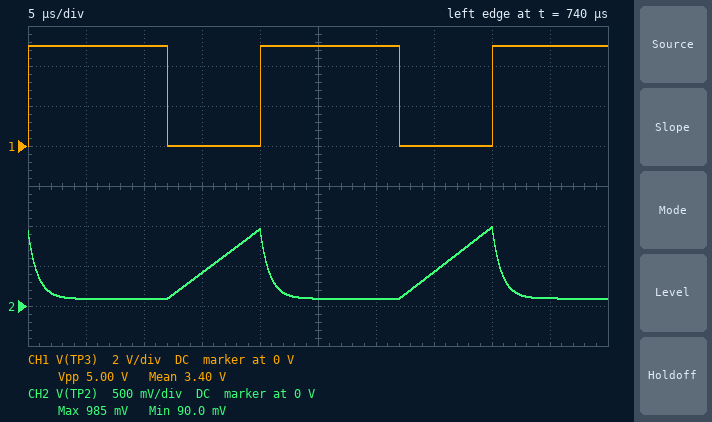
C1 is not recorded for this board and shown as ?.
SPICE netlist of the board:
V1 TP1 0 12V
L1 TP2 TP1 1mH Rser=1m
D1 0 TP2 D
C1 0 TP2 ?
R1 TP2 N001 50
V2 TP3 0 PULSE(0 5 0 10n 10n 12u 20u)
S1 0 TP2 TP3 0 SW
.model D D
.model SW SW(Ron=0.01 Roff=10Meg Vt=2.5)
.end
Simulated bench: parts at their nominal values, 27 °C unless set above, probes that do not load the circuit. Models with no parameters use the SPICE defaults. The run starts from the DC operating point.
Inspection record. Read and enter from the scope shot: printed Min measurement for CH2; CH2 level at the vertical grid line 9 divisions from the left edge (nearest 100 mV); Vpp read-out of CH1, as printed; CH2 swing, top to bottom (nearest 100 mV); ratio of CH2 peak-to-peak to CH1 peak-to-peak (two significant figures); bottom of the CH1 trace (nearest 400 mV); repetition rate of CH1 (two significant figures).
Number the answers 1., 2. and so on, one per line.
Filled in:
1. 90.0 mV
2. 100 mV
3. 5.00 V
4. 900 mV
5. 0.18
6. 0 V
7. 50 kHz
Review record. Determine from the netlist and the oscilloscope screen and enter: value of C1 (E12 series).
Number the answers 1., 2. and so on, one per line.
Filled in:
1. 82 µF
